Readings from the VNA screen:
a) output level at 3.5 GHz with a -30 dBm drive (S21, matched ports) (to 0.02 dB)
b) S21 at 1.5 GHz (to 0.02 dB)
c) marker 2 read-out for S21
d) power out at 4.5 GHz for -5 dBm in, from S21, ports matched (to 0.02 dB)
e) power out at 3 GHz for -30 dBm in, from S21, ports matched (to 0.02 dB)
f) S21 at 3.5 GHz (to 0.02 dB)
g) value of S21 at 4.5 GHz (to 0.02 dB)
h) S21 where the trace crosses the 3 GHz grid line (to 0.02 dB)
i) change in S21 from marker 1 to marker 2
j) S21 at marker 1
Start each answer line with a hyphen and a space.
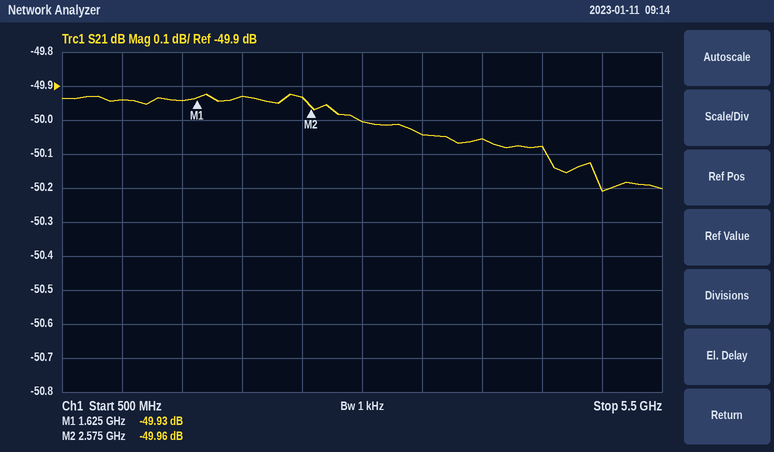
- -80.04 dBm
- -49.94 dB
- -49.96 dB
- -55.08 dBm
- -80.00 dBm
- -50.04 dB
- -50.08 dB
- -50.00 dB
- -0.03 dB
- -49.93 dB
